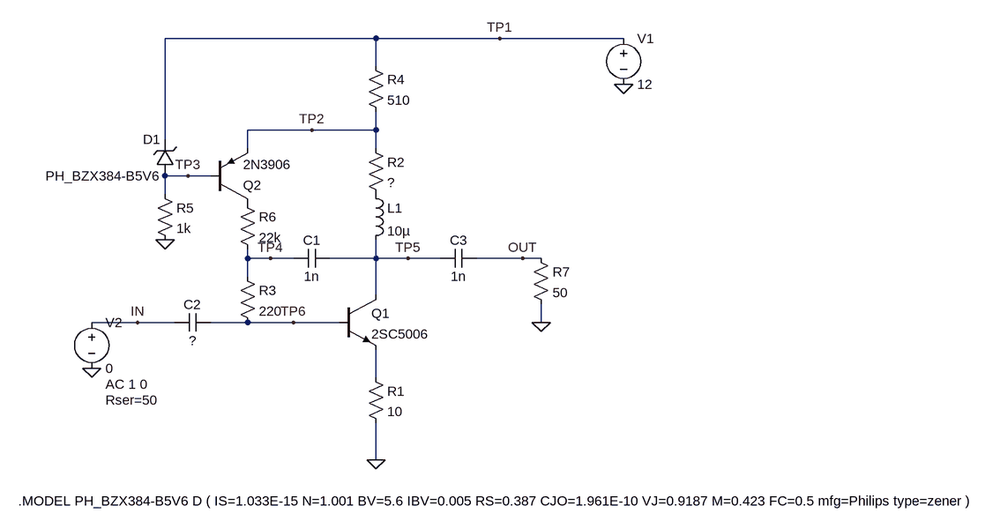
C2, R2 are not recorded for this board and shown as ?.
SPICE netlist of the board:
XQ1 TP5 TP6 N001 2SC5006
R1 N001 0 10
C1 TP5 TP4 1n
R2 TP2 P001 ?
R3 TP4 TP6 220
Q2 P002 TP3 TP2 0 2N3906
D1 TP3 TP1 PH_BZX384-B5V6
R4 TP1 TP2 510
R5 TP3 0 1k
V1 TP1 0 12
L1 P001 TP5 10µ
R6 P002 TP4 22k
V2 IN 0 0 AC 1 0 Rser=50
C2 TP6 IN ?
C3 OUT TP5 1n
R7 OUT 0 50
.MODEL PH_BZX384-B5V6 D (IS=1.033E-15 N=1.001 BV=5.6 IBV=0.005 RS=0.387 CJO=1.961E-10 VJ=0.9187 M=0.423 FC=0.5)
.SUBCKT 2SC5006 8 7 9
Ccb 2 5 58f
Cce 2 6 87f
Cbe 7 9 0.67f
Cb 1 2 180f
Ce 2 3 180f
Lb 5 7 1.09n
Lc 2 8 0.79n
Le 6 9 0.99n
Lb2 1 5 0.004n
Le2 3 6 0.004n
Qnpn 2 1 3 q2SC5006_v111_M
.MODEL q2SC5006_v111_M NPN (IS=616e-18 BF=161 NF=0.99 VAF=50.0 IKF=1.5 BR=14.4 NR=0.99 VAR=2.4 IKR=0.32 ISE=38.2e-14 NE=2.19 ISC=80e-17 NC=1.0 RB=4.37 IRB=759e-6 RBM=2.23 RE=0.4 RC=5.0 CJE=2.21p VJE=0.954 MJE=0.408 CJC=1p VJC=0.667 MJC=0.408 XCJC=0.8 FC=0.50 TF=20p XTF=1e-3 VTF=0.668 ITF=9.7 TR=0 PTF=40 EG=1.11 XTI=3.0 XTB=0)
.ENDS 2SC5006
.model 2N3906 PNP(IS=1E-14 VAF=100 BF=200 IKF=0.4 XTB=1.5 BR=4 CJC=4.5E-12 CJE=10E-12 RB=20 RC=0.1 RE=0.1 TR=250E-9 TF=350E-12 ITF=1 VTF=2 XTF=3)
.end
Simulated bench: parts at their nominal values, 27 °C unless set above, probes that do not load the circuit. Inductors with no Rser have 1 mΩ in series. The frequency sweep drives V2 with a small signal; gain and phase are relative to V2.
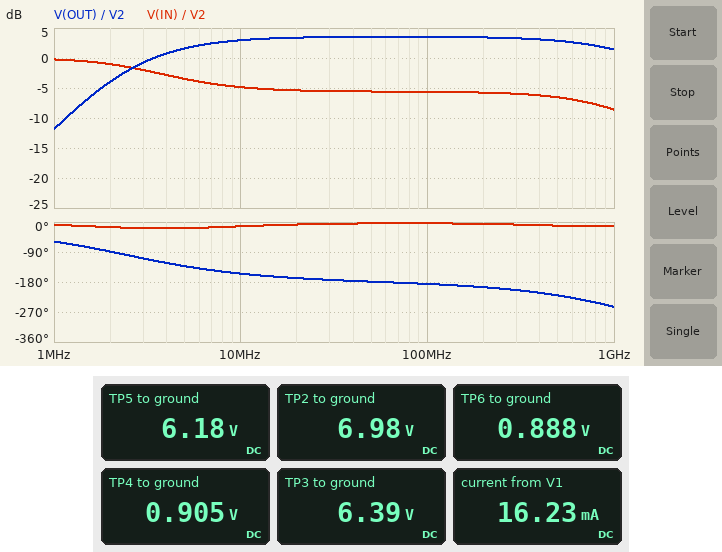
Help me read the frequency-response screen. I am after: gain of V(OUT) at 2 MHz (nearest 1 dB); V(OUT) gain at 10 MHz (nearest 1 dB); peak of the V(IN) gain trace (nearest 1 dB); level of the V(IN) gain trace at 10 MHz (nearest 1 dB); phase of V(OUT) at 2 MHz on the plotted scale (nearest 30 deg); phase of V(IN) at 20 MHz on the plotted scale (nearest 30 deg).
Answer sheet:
-4 dB
3 dB
0 dB
-5 dB
-90 deg
0 deg
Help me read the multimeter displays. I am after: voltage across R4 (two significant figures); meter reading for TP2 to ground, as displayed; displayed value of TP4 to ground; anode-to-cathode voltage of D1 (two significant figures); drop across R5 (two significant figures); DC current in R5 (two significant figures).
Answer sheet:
5.0 V
6.98 V
0.905 V
-5.6 V
6.4 V
6.4 mA
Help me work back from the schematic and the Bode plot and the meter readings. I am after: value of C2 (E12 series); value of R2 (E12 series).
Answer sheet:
470 pF
82 Ω
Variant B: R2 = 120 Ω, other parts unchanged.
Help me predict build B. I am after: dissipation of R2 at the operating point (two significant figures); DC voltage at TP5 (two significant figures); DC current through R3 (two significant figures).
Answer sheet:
11 mW
5.8 V
80 µA
